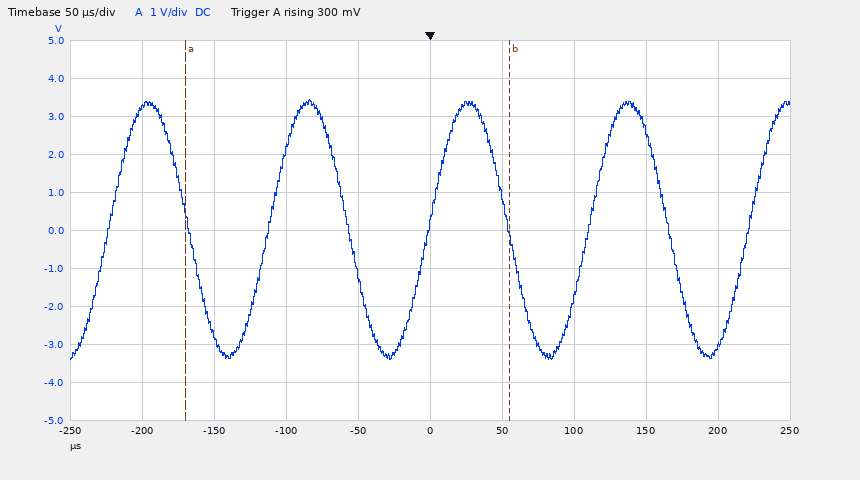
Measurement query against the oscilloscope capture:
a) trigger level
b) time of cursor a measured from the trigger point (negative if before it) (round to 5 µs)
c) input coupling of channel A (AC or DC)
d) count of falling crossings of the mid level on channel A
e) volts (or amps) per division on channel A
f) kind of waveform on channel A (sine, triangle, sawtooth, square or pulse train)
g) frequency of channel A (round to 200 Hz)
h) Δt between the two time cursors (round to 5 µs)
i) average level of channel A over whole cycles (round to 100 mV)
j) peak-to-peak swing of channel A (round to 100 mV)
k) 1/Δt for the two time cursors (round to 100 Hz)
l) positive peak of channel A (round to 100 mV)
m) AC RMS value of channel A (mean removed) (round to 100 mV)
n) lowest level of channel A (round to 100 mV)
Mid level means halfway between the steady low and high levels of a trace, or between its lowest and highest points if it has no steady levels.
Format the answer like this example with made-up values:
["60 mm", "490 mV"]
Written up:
["300 mV", "-170 µs", "DC", "4", "1 V", "sine", "9.0 kHz", "225 µs", "0.0 V", "6.8 V", "4.4 kHz", "3.4 V", "2.4 V", "-3.4 V"]
